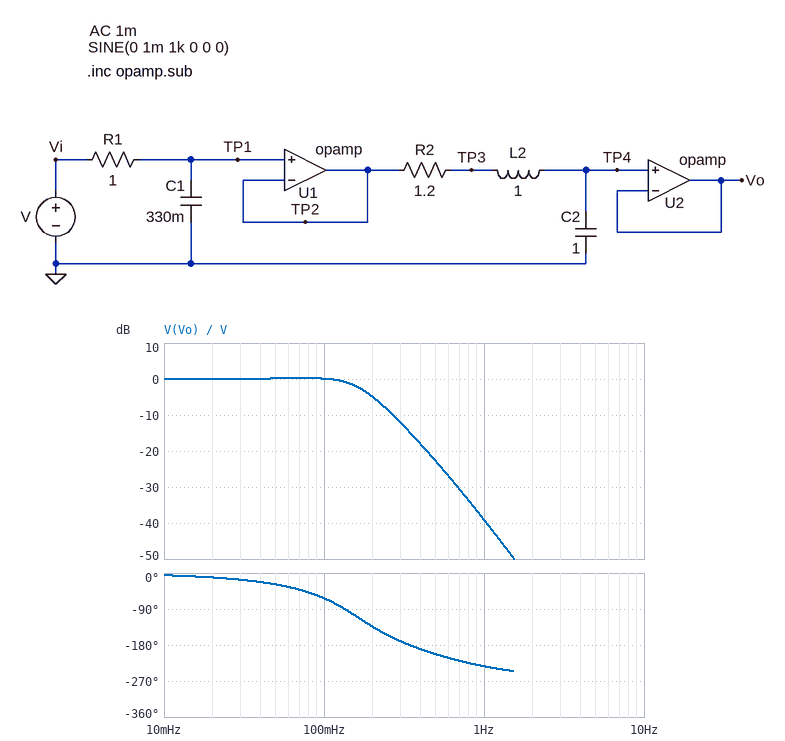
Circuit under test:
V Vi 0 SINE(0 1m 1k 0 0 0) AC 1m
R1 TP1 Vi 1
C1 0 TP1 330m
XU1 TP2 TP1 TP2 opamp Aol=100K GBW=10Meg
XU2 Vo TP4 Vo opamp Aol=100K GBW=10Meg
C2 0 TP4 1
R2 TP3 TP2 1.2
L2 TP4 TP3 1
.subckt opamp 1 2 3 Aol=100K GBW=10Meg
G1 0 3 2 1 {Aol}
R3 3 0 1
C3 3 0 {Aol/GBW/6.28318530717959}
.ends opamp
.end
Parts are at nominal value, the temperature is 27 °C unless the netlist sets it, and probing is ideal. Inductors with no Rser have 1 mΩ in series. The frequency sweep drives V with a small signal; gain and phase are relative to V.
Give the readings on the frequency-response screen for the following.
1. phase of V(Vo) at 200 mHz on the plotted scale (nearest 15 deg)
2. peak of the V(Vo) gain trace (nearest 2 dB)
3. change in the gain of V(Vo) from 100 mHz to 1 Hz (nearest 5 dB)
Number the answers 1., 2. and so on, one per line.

1. -135 deg
2. 0 dB
3. -40 dB
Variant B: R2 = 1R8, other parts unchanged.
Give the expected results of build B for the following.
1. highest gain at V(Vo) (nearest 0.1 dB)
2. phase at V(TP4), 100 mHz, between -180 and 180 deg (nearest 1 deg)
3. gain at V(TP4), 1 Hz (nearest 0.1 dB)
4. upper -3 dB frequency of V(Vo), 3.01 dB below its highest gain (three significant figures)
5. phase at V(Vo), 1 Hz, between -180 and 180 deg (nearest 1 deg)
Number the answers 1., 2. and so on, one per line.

1. 0 dB
2. -74 deg
3. -39.3 dB
4. 114 mHz
5. 132 deg
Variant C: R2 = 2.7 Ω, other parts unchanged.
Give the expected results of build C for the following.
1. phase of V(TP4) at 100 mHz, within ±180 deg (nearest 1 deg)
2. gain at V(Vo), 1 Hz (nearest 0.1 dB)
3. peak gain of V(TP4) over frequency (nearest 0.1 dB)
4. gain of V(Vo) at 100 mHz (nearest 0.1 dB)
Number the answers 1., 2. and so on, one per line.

1. -82 deg
2. -39.7 dB
3. 0 dB
4. -5.3 dB
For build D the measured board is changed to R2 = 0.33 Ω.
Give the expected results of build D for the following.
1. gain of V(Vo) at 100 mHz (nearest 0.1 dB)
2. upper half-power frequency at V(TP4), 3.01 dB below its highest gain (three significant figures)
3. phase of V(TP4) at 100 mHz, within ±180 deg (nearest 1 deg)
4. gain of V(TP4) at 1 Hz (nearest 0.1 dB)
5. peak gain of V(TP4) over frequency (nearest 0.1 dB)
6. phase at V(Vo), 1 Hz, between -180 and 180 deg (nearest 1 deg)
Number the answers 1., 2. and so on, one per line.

1. 3.7 dB
2. 179 mHz
3. -31 deg
4. -39.0 dB
5. 9.3 dB
6. 119 deg
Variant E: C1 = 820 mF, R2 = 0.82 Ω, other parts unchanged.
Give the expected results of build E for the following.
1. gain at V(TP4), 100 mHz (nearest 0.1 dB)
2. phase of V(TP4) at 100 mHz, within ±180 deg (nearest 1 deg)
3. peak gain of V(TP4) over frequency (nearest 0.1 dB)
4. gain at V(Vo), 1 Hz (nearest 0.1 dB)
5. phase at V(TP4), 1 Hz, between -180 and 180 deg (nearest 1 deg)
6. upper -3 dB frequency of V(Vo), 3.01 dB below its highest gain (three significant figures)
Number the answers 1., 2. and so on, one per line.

1. 1.0 dB
2. -68 deg
3. 1.1 dB
4. -46.2 dB
5. 109 deg
6. 175 mHz
